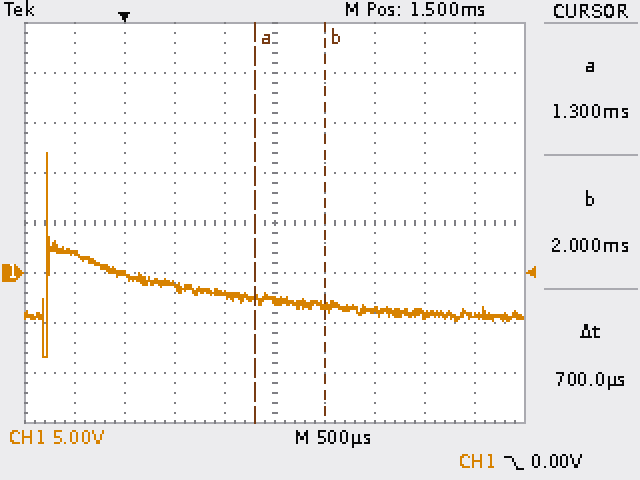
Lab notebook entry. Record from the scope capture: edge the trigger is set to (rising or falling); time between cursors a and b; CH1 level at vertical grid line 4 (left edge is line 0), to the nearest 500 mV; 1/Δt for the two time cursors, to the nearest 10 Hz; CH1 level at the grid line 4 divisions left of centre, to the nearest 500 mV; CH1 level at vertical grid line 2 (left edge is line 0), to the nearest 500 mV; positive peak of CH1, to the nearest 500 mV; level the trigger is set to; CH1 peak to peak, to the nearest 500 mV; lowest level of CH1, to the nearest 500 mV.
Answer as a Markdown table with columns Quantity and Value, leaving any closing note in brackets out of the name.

| Quantity | Value |
|---|---|
| edge the trigger is set to | falling |
| time between cursors a and b | 700 µs |
| CH1 level at vertical grid line 4 (left edge is line 0), to the nearest 500 mV | -2.0 V |
| 1/Δt for the two time cursors, to the nearest 10 Hz | 1.43 kHz |
| CH1 level at the grid line 4 divisions left of centre, to the nearest 500 mV | 2.0 V |
| CH1 level at vertical grid line 2 (left edge is line 0), to the nearest 500 mV | 0.0 V |
| positive peak of CH1, to the nearest 500 mV | 12.0 V |
| level the trigger is set to | 0.00 V |
| CH1 peak to peak, to the nearest 500 mV | 20.5 V |
| lowest level of CH1, to the nearest 500 mV | -8.5 V |
